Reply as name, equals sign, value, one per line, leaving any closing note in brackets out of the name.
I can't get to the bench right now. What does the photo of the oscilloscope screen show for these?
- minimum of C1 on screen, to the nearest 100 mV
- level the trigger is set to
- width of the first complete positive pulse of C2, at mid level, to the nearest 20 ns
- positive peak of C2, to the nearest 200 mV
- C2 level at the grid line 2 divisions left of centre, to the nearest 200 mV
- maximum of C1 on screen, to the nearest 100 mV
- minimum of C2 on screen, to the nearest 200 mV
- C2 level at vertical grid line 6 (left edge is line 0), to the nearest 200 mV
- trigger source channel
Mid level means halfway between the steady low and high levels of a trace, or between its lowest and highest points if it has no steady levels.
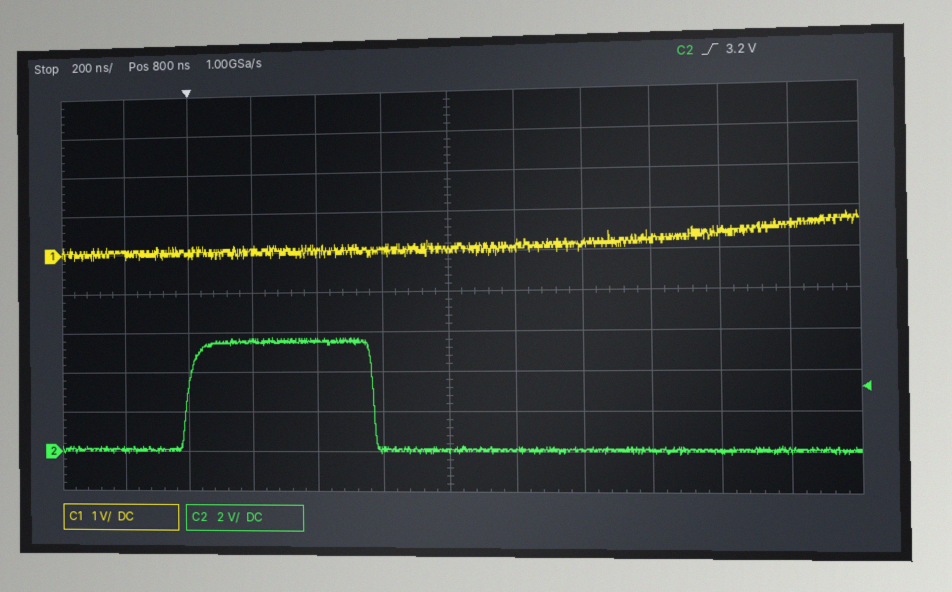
minimum of C1 on screen, to the nearest 100 mV = -100 mV
level the trigger is set to = 3.2 V
width of the first complete positive pulse of C2, at mid level, to the nearest 20 ns = 580 ns
positive peak of C2, to the nearest 200 mV = 5.8 V
C2 level at the grid line 2 divisions left of centre, to the nearest 200 mV = 5.6 V
maximum of C1 on screen, to the nearest 100 mV = 800 mV
minimum of C2 on screen, to the nearest 200 mV = -200 mV
C2 level at vertical grid line 6 (left edge is line 0), to the nearest 200 mV = 0.0 V
trigger source channel = C2
